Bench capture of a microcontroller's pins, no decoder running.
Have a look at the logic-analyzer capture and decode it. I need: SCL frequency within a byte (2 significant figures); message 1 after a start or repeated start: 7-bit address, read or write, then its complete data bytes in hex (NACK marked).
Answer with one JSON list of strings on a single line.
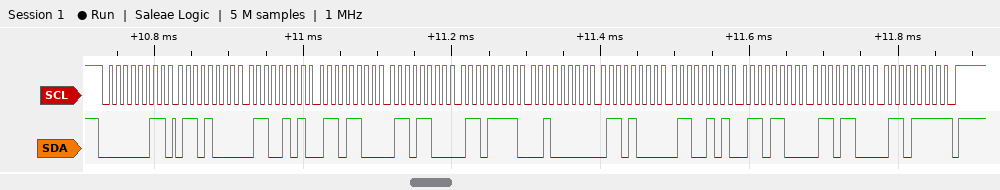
["100 kHz", "0x01 read: 68 65 6C 6C 6F 20 68 65 6C 6C 6F NACK"]
